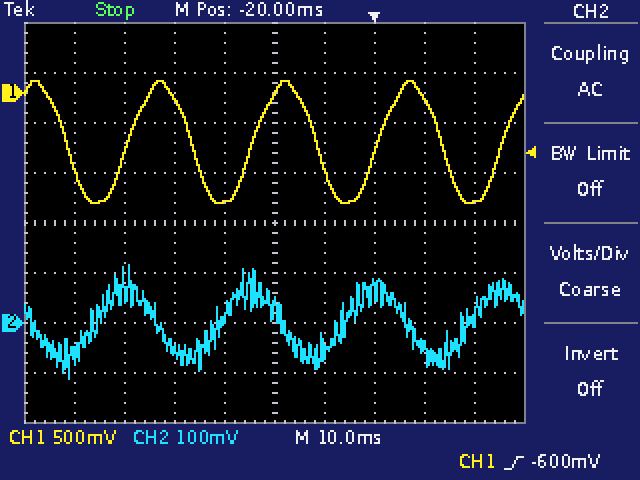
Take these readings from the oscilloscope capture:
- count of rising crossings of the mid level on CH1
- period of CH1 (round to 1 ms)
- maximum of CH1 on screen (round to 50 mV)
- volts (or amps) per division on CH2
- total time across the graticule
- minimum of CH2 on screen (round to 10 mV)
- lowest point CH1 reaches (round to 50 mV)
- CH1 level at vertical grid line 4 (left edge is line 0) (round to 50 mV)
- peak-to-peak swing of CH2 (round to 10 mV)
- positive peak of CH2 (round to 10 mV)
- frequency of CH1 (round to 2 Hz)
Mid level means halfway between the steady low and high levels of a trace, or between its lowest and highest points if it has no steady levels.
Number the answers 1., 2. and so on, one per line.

1. 4
2. 25 ms
3. 100 mV
4. 100 mV
5. 100 ms
6. -110 mV
7. -1.10 V
8. -1.10 V
9. 230 mV
10. 120 mV
11. 40 Hz
